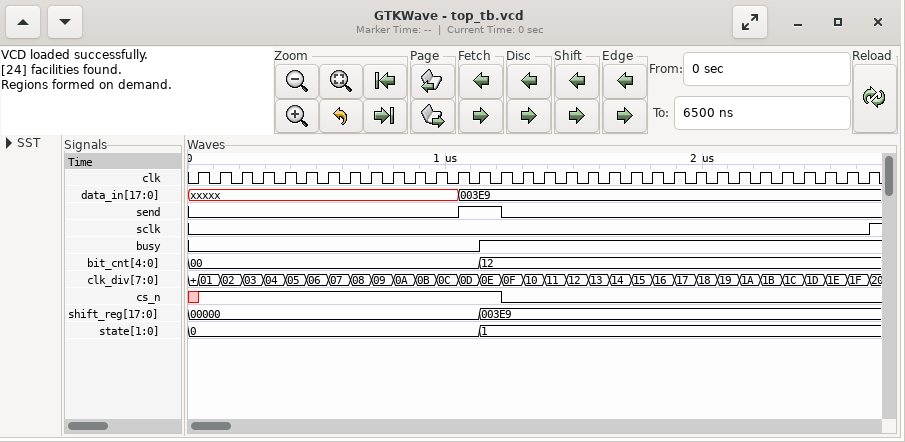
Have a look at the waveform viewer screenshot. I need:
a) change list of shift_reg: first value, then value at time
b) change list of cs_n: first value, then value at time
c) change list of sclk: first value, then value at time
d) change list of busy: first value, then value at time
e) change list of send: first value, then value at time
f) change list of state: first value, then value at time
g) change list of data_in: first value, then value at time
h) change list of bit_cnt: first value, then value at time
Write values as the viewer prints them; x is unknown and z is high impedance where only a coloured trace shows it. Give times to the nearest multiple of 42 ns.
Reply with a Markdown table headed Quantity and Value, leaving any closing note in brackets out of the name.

| Quantity | Value |
|---|---|
| change list of shift_reg: first value, then value at time | 00000, 003E9 at 1134 ns |
| change list of cs_n: first value, then value at time | x, 1 at 42 ns, 0 at 1218 ns |
| change list of sclk: first value, then value at time | 0, 1 at 2646 ns |
| change list of busy: first value, then value at time | 0, 1 at 1134 ns |
| change list of send: first value, then value at time | 0, 1 at 1050 ns, 0 at 1218 ns |
| change list of state: first value, then value at time | 0, 1 at 1134 ns |
| change list of data_in: first value, then value at time | xxxxx, 003E9 at 1050 ns |
| change list of bit_cnt: first value, then value at time | 00, 12 at 1134 ns |
